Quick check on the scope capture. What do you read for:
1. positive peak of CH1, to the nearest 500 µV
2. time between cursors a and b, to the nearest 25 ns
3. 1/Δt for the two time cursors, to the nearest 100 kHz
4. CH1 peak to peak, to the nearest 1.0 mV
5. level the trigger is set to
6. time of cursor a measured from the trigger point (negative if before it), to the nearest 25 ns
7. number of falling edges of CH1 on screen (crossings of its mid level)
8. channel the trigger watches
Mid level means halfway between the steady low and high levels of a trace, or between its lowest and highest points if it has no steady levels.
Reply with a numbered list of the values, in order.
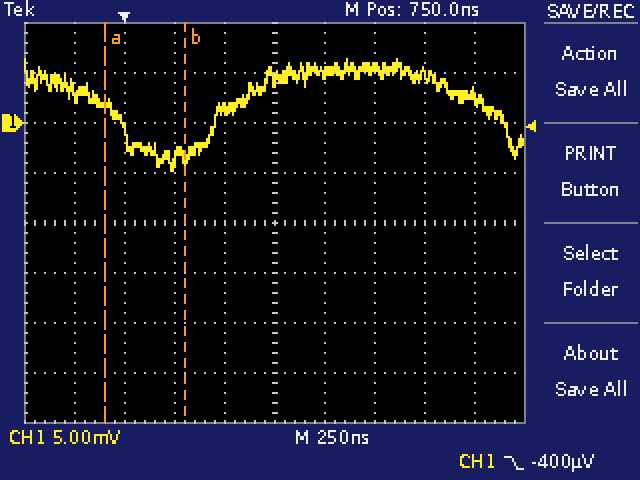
1. 6.5 mV
2. 400 ns
3. 2.5 MHz
4. 11.0 mV
5. -400 µV
6. -100 ns
7. 2
8. CH1
